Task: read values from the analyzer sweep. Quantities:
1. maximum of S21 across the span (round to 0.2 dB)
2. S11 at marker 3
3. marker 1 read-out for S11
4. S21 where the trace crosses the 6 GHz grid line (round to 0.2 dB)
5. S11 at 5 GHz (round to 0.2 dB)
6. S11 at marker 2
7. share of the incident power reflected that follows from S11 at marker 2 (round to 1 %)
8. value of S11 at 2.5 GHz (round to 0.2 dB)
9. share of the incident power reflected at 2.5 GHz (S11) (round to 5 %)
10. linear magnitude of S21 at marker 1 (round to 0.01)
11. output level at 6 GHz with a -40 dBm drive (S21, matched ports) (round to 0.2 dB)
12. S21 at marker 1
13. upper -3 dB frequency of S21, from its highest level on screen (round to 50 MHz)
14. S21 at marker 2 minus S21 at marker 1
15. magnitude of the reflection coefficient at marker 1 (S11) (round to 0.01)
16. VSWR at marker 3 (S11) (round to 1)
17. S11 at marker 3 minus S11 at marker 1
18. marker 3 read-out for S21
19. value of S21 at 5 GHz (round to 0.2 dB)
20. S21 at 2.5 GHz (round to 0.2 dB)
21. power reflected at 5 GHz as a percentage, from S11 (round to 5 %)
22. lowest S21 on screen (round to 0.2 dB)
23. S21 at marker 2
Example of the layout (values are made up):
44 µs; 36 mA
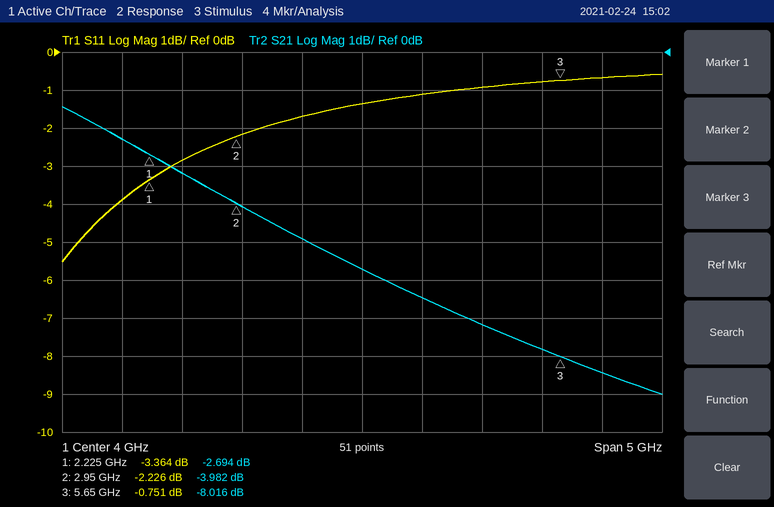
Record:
-1.4 dB; -0.751 dB; -3.364 dB; -8.4 dB; -1.0 dB; -2.226 dB; 60 %; -2.8 dB; 50 %; 0.73; -48.4 dBm; -2.694 dB; 3.20 GHz; -1.288 dB; 0.68; 23; 2.613 dB; -8.016 dB; -7.2 dB; -3.2 dB; 80 %; -9.0 dB; -3.982 dB
